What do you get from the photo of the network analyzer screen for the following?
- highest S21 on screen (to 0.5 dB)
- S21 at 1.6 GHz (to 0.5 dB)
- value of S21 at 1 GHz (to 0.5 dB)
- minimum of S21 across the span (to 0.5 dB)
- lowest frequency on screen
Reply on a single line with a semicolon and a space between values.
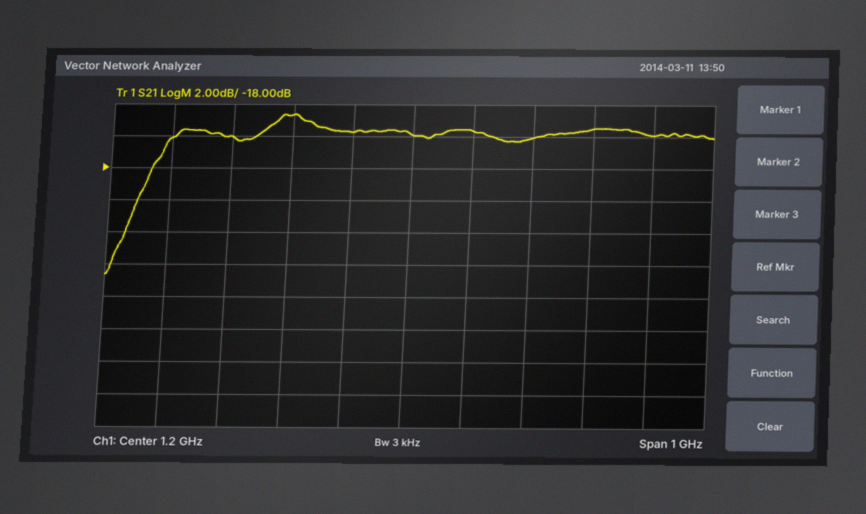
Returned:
-14.5 dB; -16.0 dB; -14.5 dB; -24.5 dB; 700 MHz
